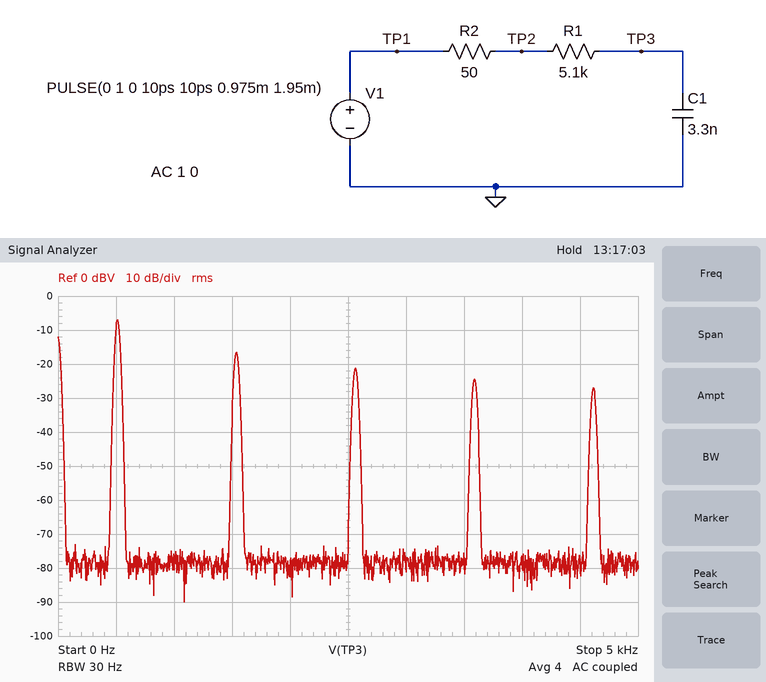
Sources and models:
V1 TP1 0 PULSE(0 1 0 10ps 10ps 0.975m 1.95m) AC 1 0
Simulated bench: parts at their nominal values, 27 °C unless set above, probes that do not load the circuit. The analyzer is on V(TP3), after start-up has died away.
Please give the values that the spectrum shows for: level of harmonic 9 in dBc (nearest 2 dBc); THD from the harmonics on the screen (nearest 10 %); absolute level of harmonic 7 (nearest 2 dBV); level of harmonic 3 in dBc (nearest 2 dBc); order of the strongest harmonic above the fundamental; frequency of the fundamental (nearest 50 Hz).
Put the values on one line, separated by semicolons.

-20 dBc; 40 %; -24 dBV; -10 dBc; 3; 500 Hz
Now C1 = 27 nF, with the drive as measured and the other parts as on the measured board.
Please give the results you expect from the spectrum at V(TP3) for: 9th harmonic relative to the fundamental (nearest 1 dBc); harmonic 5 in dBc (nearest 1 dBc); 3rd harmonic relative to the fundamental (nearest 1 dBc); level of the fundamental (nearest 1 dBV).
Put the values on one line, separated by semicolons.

-31 dBc; -21 dBc; -13 dBc; -8 dBV
